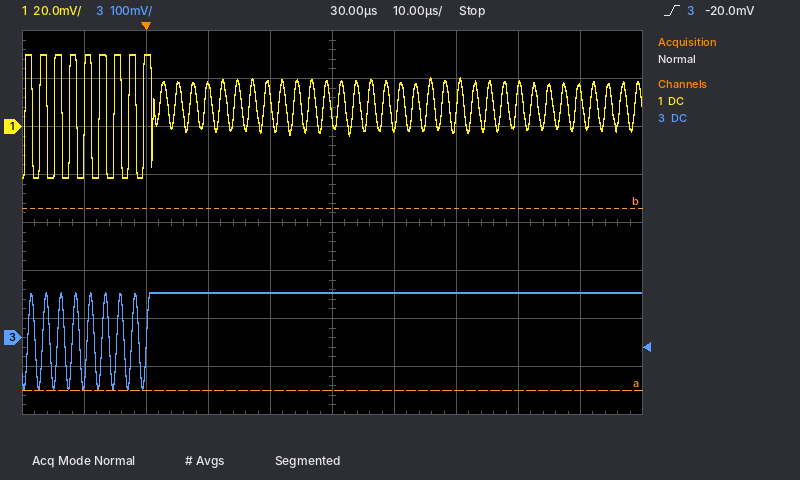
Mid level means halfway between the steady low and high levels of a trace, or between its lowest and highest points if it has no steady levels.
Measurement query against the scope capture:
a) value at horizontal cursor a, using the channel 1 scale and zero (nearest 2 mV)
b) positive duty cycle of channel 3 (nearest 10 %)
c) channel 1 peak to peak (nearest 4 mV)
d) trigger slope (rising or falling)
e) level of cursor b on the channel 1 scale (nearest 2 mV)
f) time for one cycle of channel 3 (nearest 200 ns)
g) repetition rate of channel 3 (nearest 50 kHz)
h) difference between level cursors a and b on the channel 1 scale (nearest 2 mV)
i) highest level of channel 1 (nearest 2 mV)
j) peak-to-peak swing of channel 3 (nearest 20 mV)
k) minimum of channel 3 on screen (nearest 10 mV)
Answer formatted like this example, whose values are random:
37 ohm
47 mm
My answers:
-110 mV
50 %
52 mV
rising
-34 mV
2.4 µs
400 kHz
76 mV
30 mV
200 mV
-110 mV
